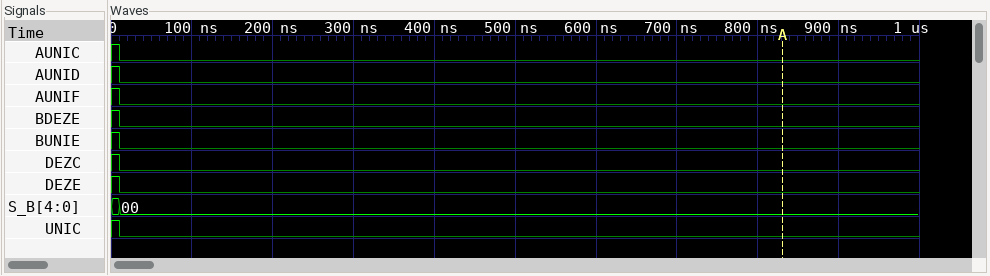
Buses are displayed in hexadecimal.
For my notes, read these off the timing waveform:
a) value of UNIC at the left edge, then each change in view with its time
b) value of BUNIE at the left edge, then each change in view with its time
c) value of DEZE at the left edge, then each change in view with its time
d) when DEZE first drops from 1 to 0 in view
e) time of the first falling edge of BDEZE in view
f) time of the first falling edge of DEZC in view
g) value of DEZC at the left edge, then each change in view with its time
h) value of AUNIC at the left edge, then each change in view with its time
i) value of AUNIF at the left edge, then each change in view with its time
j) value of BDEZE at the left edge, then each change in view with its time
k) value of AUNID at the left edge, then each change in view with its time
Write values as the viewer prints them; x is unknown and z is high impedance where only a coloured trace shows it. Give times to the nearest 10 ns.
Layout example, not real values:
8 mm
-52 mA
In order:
1, 0 at 10 ns
1, 0 at 10 ns
1, 0 at 10 ns
10 ns
10 ns
10 ns
1, 0 at 10 ns
1, 0 at 10 ns
1, 0 at 10 ns
1, 0 at 10 ns
1, 0 at 10 ns
